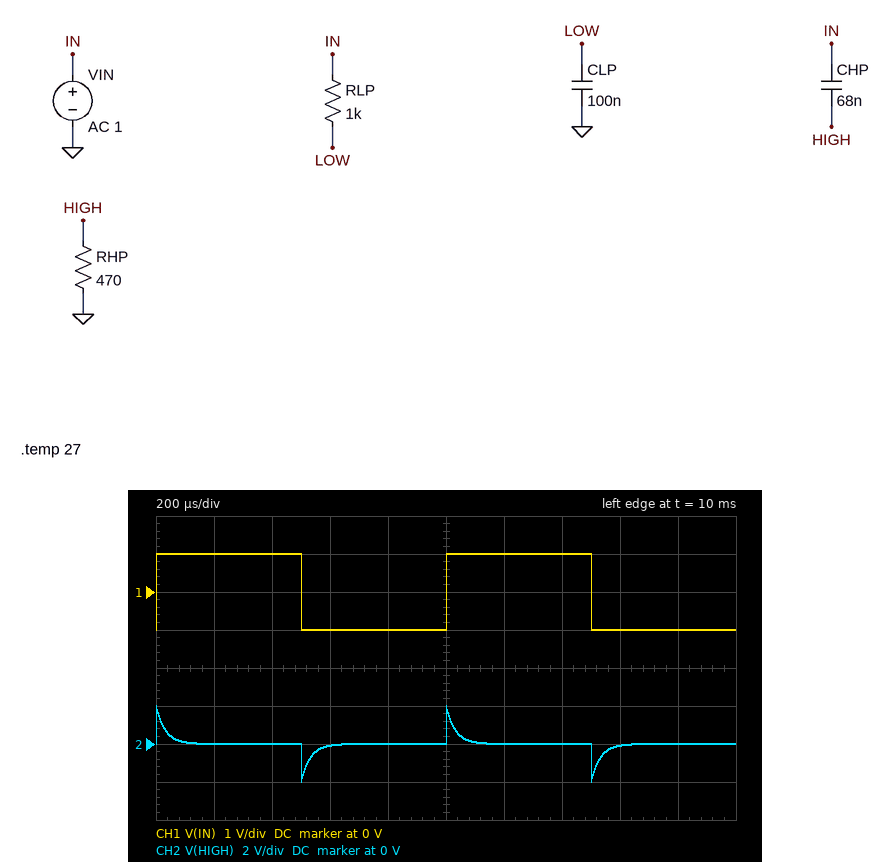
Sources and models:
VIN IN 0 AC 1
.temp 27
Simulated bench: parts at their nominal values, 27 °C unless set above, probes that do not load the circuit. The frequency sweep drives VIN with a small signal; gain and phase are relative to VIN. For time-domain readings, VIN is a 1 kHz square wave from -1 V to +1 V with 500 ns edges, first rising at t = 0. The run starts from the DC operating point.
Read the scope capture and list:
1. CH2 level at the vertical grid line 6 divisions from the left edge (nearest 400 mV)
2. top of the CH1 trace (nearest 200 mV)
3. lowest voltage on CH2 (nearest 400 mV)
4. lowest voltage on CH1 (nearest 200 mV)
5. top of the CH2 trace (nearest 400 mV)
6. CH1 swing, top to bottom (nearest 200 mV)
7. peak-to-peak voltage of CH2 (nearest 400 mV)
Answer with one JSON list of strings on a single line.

["0 V", "1.0 V", "-2.0 V", "-1.0 V", "2.0 V", "2.0 V", "4.0 V"]
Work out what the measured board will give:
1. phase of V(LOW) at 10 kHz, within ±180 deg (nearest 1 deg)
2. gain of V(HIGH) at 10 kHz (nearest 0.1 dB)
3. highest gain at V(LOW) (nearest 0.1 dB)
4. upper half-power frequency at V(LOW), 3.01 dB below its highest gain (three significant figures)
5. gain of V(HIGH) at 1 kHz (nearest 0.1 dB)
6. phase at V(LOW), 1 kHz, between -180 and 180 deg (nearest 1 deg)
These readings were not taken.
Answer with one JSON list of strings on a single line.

["-81 deg", "-1.0 dB", "0 dB", "1.59 kHz", "-14.1 dB", "-32 deg"]
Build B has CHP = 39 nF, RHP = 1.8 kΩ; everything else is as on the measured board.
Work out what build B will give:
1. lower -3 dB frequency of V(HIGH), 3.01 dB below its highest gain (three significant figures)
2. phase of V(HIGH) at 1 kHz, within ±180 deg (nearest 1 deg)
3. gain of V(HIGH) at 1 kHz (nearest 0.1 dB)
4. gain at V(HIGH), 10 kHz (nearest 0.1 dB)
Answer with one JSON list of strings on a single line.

["2.27 kHz", "66 deg", "-7.9 dB", "-0.2 dB"]
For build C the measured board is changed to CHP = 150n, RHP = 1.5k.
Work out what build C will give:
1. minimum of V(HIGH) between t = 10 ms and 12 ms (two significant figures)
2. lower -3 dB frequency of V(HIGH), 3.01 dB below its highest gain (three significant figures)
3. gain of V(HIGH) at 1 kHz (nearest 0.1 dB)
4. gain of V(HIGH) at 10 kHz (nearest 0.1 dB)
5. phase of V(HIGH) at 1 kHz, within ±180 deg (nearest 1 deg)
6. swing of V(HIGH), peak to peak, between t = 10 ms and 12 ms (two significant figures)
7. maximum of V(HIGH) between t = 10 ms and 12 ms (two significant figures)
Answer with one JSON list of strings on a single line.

["-1.8 V", "707 Hz", "-1.8 dB", "0 dB", "35 deg", "3.6 V", "1.8 V"]
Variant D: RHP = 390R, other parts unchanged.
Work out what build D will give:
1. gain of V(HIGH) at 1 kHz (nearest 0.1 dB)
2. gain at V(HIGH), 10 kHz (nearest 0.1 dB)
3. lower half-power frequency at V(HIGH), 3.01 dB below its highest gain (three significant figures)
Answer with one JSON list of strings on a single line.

["-15.7 dB", "-1.3 dB", "6.00 kHz"]
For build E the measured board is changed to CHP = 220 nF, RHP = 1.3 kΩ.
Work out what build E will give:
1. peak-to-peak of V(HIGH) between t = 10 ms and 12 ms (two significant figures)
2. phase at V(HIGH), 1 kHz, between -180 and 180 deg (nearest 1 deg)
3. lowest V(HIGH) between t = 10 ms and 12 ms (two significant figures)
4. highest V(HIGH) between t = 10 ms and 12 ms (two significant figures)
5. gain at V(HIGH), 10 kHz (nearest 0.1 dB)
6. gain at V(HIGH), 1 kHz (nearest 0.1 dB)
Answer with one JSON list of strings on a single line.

["3.4 V", "29 deg", "-1.7 V", "1.7 V", "0 dB", "-1.2 dB"]
